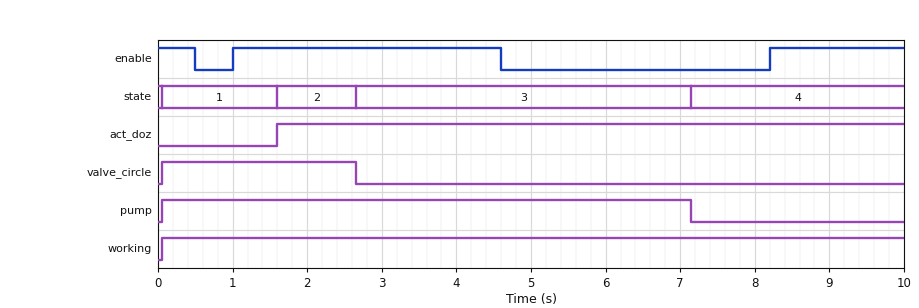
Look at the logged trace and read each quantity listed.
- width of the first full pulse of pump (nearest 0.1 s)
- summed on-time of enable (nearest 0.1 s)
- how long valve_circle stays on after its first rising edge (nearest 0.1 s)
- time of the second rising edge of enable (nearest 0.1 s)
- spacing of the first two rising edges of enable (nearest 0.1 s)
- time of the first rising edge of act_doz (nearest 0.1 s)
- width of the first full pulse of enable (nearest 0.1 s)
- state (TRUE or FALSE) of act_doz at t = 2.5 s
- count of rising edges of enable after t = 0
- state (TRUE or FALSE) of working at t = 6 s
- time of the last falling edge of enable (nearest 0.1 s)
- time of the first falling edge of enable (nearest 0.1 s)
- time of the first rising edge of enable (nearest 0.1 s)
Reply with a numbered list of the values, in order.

1. 7.1 s
2. 5.9 s
3. 2.6 s
4. 8.2 s
5. 7.2 s
6. 1.6 s
7. 3.6 s
8. TRUE
9. 2
10. TRUE
11. 4.6 s
12. 0.5 s
13. 1.0 s
